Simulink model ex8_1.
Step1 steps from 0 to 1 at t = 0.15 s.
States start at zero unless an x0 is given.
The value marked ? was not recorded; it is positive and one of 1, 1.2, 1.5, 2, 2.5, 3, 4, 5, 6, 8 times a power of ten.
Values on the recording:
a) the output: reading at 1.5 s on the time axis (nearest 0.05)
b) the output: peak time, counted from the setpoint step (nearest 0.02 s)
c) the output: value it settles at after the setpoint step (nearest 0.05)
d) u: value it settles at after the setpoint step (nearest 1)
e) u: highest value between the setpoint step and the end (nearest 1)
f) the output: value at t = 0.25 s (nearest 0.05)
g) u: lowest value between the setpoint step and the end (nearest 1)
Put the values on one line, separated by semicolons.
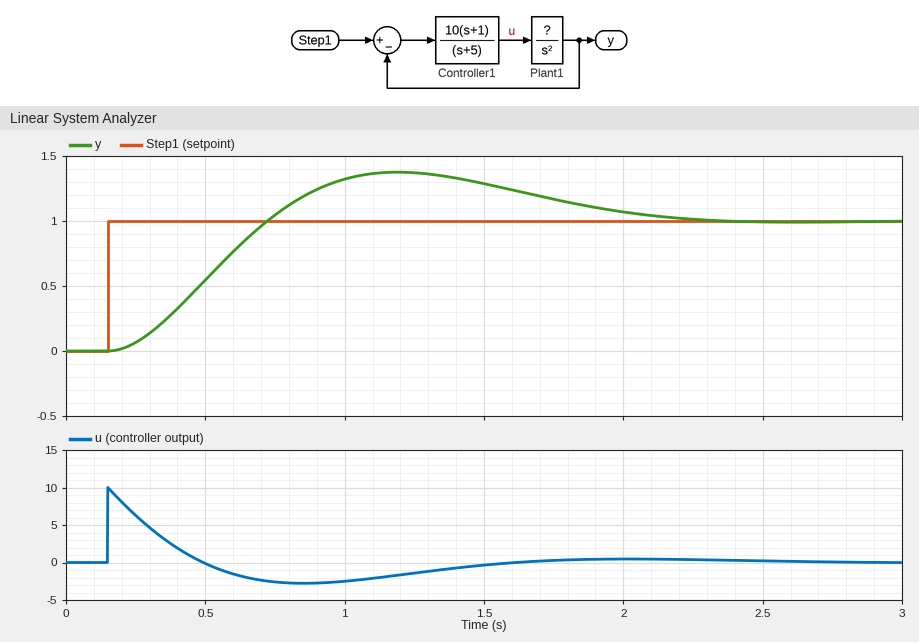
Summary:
1.30; 1.04 s; 1.00; 0; 10; 0.05; -3
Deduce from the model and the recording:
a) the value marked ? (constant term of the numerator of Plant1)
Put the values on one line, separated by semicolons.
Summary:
1.5
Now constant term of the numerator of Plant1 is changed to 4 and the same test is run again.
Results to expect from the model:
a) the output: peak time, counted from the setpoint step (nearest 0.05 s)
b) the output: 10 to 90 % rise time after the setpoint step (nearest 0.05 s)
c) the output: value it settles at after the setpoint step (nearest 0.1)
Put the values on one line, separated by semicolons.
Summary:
0.55 s; 0.20 s; 1.0
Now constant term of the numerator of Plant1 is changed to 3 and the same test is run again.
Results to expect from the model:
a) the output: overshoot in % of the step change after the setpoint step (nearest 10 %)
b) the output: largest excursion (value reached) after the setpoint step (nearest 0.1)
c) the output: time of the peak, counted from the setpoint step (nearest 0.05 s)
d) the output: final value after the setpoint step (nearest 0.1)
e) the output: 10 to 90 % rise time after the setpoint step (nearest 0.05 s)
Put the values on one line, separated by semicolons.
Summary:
40 %; 1.4; 0.65 s; 1.0; 0.25 s
